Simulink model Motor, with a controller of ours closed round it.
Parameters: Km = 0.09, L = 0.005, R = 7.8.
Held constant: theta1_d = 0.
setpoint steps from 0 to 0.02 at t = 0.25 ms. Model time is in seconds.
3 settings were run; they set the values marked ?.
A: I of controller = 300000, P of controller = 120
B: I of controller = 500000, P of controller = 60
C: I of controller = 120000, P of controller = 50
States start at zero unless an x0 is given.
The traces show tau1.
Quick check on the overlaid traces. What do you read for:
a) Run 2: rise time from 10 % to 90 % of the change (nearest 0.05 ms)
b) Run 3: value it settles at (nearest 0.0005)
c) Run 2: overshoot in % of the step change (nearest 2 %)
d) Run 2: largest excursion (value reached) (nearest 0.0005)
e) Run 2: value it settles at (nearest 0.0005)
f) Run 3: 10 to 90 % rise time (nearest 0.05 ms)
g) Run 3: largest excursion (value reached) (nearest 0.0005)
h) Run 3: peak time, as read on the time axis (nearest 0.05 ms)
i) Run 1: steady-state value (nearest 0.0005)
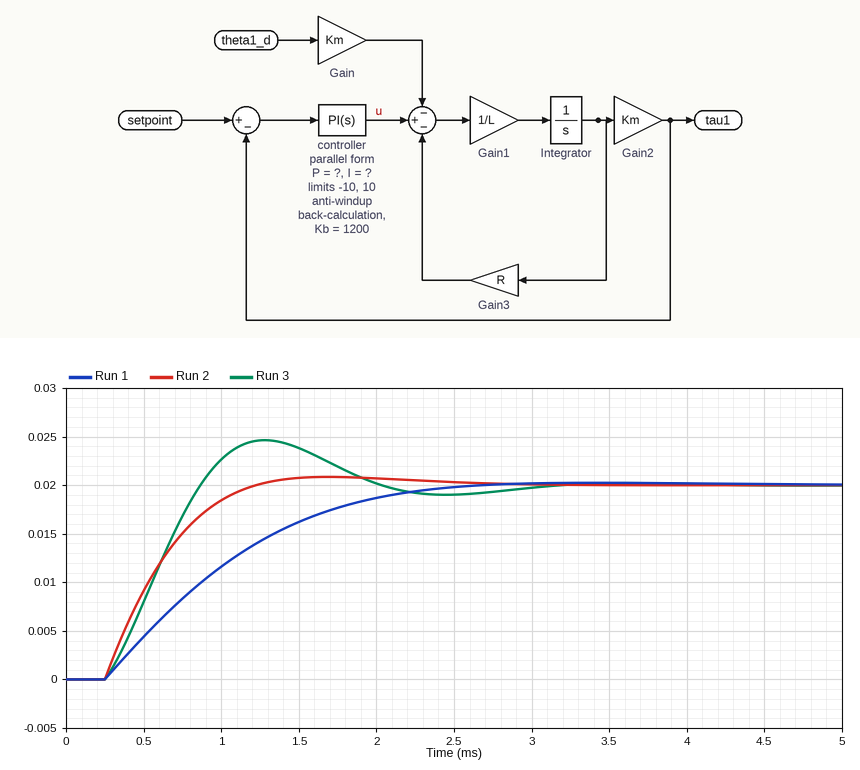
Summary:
0.65 ms
0.0200
4 %
0.0210
0.0200
0.45 ms
0.0245
1.30 ms
0.0200
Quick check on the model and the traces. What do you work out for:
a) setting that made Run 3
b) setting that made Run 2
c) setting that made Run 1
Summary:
B
A
C
